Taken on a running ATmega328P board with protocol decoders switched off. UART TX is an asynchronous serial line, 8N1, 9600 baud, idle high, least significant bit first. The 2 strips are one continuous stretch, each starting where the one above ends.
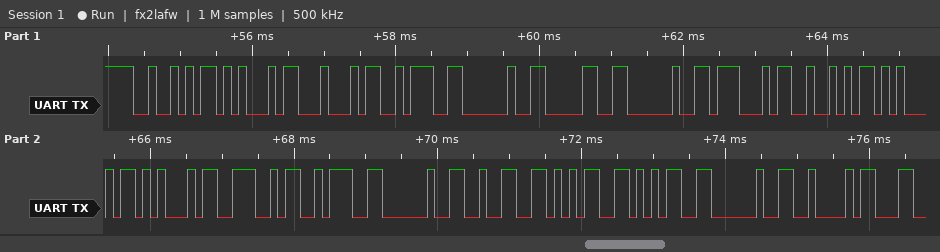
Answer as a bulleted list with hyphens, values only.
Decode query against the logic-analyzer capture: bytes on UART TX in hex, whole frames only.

- 52 45 44 3A 20 30 20 47 52 45 45 4E 3A 20 32 35 35 20 42
